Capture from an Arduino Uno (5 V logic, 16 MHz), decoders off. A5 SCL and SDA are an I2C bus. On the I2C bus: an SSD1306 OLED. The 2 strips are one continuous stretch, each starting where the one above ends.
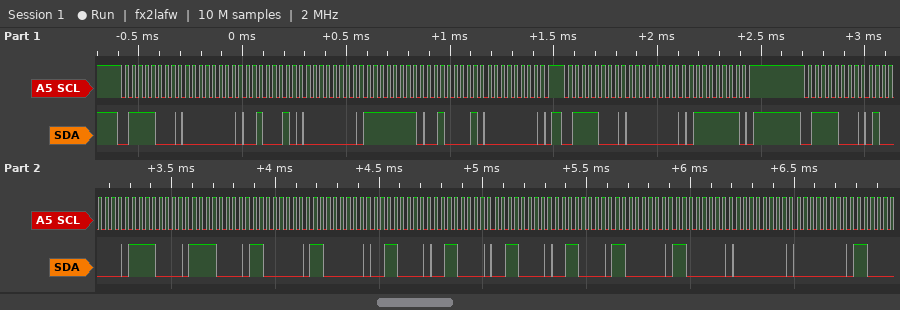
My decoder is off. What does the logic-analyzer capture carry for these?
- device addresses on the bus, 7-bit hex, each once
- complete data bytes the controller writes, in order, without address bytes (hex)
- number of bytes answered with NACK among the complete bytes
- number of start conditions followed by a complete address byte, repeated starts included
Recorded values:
0x3C
00 22 00 FF 21 00 00 7F 40 F0 F0 C0 C0 30 30 30 30 C0 C0 00 00
0
3
